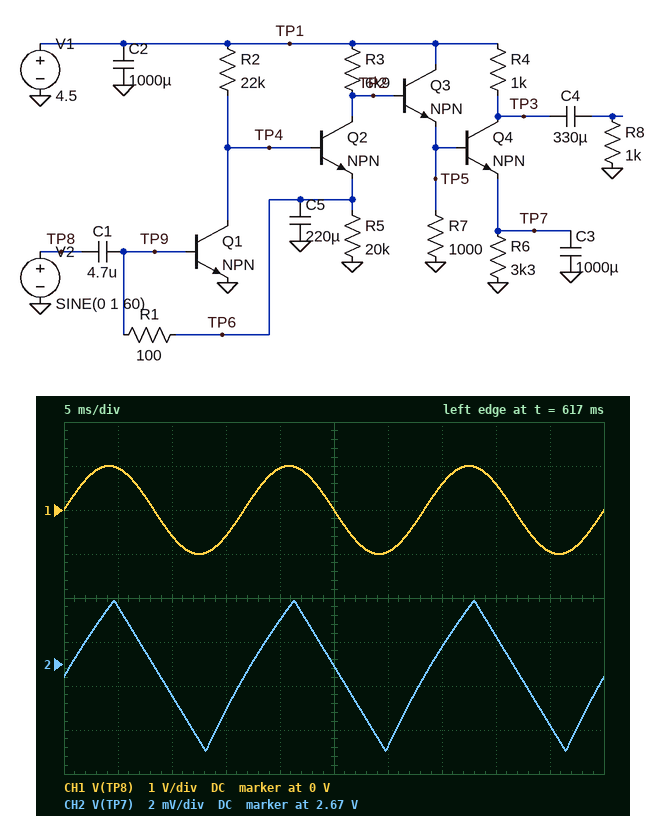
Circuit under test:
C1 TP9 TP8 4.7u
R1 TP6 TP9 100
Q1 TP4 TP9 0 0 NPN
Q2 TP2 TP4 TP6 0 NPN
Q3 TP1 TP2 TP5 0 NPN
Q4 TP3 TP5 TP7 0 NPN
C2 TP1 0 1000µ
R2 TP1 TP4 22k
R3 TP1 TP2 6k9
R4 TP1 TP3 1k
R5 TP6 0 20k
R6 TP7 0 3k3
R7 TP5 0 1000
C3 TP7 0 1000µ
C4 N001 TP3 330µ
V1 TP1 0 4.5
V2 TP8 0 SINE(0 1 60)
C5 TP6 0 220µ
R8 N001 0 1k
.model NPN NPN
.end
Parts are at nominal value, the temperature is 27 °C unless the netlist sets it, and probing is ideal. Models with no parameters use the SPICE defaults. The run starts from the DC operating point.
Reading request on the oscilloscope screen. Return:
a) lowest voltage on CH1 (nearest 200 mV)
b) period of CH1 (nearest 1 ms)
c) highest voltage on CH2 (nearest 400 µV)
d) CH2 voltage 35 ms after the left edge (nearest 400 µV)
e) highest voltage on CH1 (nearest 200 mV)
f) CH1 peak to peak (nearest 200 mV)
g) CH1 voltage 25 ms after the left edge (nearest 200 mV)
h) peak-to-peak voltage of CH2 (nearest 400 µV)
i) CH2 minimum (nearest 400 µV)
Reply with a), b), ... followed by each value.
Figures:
a) -1.0 V
b) 17 ms
c) 2.6728 V
d) 2.6708 V
e) 1.0 V
f) 2.0 V
g) 0 V
h) 6.8 mV
i) 2.6660 V
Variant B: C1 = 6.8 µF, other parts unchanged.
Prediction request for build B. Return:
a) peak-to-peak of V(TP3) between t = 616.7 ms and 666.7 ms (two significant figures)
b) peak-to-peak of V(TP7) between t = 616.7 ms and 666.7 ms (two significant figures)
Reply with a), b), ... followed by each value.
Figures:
a) 1.1 V
b) 7.6 mV
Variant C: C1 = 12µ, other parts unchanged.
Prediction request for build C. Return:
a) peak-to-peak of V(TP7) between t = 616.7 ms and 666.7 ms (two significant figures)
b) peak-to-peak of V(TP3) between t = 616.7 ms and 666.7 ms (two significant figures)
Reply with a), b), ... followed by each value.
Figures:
a) 8.7 mV
b) 1.3 V
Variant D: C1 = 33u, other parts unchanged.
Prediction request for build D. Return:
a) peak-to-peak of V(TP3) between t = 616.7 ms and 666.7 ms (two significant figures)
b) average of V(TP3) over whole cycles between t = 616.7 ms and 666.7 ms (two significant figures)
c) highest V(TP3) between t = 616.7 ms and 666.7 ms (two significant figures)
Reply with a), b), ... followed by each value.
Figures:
a) 1.5 V
b) 3.8 V
c) 4.1 V
